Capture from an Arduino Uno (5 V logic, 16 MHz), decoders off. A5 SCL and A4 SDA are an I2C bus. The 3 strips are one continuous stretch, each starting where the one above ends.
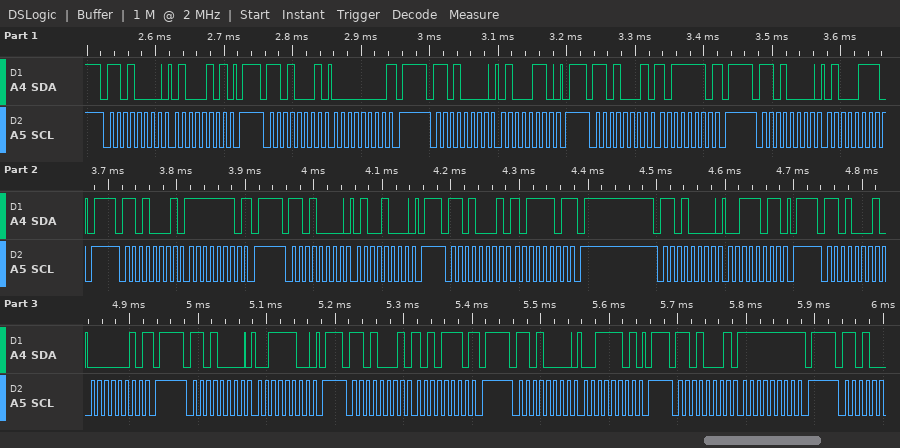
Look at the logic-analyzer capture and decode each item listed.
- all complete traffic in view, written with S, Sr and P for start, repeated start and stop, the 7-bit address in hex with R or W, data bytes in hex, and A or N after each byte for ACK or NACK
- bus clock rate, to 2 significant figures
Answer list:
S 68W A 45 A P S 68R A 00 N P S 68W A 46 A P S 68R A BE N P S 68W A 47 A P S 68R A FE N P S 68W A 48 A P S 68R A BD N P S 68W A 3B A P S 68R A 02 N P S 68W A 3C A P S 68R A AE N P S 68W A 3D A P S 68R A FF N P
100 kHz
